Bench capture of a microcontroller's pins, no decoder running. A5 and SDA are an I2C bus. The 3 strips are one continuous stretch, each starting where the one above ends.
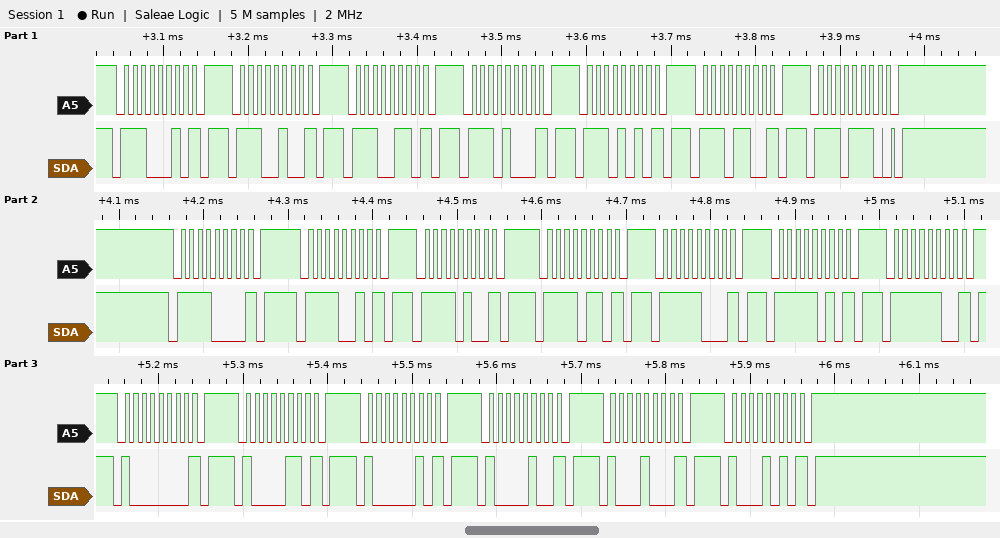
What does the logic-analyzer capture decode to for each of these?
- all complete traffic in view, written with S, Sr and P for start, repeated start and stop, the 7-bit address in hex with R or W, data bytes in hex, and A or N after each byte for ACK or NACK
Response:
S 71W N P S 72W N P S 73W N P S 74W N P S 75W N P S 76W N P S 77W A P S 78W N P S 79W N P S 7AW N P S 7BW N P S 7CW N P S 7DW N P S 7EW N P S 40W N P S 43W N P S 41W N P S 42W N P S 44W N P S 45W N P
